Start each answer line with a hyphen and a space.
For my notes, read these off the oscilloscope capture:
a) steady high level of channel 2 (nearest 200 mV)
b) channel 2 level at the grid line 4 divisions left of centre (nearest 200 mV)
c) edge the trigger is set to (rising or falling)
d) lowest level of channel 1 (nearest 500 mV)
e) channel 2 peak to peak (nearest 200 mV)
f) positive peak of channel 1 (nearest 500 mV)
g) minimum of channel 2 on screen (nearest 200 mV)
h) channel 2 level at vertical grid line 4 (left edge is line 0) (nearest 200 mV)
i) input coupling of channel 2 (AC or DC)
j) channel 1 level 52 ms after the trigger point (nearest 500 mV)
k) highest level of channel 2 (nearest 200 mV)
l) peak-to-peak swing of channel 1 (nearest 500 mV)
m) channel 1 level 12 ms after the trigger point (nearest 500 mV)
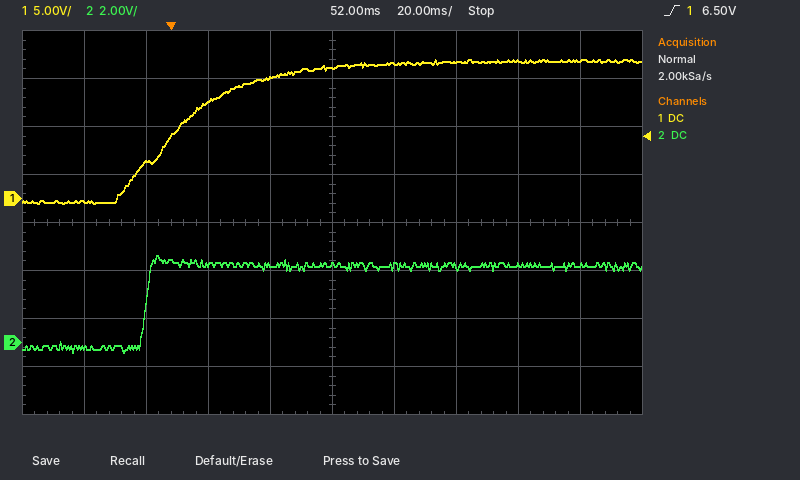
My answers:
- 3.2 V
- -200 mV
- rising
- -500 mV
- 4.0 V
- 14.5 V
- -400 mV
- 3.2 V
- DC
- 13.5 V
- 3.6 V
- 15.0 V
- 10.0 V
